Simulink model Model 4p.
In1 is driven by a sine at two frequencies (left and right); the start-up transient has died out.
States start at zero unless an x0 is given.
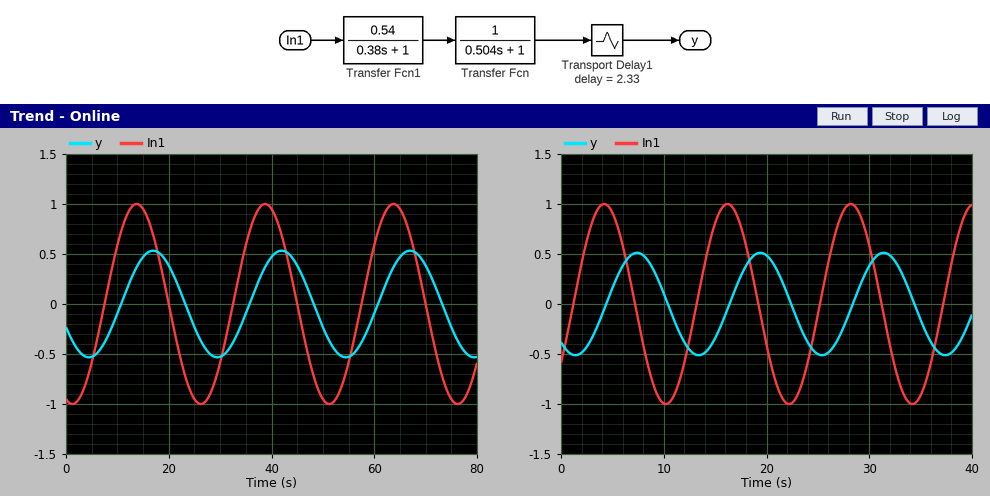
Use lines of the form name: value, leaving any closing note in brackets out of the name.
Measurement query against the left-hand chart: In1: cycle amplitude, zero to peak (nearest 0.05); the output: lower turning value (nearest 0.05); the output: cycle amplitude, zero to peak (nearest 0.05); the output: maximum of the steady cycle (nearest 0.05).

In1: cycle amplitude, zero to peak: 1.00
the output: lower turning value: -0.55
the output: cycle amplitude, zero to peak: 0.55
the output: maximum of the steady cycle: 0.55
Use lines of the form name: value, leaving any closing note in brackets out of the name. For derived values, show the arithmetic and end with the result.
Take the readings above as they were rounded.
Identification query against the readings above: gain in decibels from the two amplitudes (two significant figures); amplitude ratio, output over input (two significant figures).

gain in decibels from the two amplitudes: 20 log10(0.55 / 1) = -5.2 dB
amplitude ratio, output over input: 0.55 / 1 = 0.55
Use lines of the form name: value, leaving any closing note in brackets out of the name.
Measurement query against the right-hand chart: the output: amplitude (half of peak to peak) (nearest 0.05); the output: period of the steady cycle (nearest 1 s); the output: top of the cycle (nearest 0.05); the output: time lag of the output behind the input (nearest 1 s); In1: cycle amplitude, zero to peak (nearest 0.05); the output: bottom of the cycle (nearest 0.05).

the output: amplitude (half of peak to peak): 0.50
the output: period of the steady cycle: 12 s
the output: top of the cycle: 0.50
the output: time lag of the output behind the input: 3 s
In1: cycle amplitude, zero to peak: 1.00
the output: bottom of the cycle: -0.50
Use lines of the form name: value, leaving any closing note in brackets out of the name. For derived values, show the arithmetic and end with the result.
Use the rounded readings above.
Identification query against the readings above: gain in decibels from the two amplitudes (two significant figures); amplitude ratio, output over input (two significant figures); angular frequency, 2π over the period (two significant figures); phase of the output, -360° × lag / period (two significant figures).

gain in decibels from the two amplitudes: 20 log10(0.5 / 1) = -6.0 dB
amplitude ratio, output over input: 0.5 / 1 = 0.50
angular frequency, 2π over the period: 2π / 12 = 0.52 rad/s
phase of the output, -360° × lag / period: -360 × 3 / 12 = -90°
